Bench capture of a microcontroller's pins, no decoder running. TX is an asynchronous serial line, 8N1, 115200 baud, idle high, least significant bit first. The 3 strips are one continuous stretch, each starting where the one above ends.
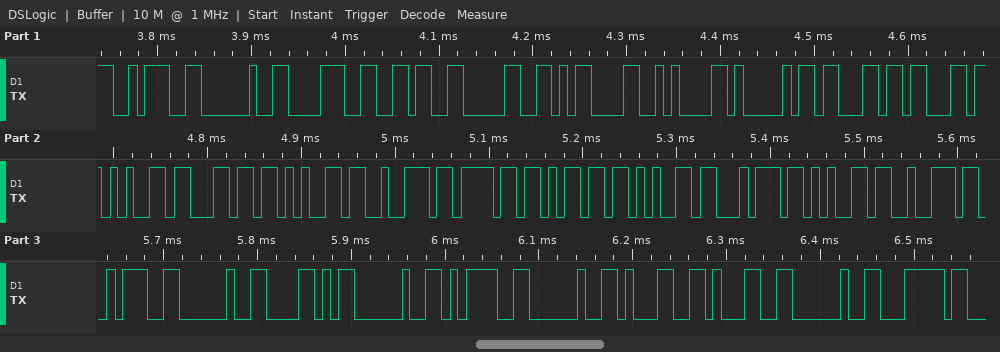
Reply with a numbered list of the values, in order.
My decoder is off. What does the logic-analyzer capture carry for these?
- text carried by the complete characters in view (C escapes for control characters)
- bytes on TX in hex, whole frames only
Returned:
1. ": 860\r\nAccelerometer: X = 11 |"
2. 0x3A 0x20 0x38 0x36 0x30 0x0D 0x0A 0x41 0x63 0x63 0x65 0x6C 0x65 0x72 0x6F 0x6D 0x65 0x74 0x65 0x72 0x3A 0x20 0x58 0x20 0x3D 0x20 0x31 0x31 0x20 0x7C
